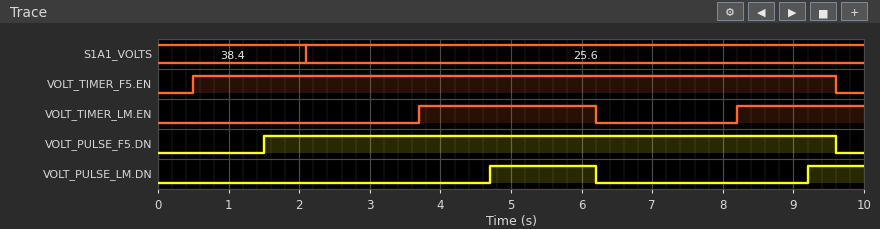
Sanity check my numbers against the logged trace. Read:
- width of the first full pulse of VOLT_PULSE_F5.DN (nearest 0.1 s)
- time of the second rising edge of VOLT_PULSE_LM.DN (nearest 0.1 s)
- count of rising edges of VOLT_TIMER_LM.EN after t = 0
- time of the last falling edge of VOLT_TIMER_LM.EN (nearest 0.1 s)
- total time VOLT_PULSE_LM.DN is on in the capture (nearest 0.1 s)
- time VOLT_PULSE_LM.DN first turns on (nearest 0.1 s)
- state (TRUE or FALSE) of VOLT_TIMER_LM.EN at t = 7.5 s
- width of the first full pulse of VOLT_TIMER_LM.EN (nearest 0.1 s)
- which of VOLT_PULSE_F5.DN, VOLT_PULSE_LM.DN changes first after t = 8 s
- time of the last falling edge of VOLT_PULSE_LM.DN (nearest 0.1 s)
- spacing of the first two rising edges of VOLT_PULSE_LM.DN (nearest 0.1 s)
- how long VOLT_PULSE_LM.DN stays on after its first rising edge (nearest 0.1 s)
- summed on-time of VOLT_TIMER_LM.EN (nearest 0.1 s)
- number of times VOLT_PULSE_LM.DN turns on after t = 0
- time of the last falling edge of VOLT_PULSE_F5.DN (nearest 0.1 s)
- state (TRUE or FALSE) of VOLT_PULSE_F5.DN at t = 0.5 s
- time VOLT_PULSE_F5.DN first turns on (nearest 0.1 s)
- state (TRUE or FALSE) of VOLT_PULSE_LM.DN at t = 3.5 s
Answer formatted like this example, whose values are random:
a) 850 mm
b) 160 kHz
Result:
a) 8.1 s
b) 9.2 s
c) 2
d) 6.2 s
e) 2.3 s
f) 4.7 s
g) FALSE
h) 2.5 s
i) VOLT_PULSE_LM.DN
j) 6.2 s
k) 4.5 s
l) 1.5 s
m) 4.3 s
n) 2
o) 9.6 s
p) FALSE
q) 1.5 s
r) FALSE
